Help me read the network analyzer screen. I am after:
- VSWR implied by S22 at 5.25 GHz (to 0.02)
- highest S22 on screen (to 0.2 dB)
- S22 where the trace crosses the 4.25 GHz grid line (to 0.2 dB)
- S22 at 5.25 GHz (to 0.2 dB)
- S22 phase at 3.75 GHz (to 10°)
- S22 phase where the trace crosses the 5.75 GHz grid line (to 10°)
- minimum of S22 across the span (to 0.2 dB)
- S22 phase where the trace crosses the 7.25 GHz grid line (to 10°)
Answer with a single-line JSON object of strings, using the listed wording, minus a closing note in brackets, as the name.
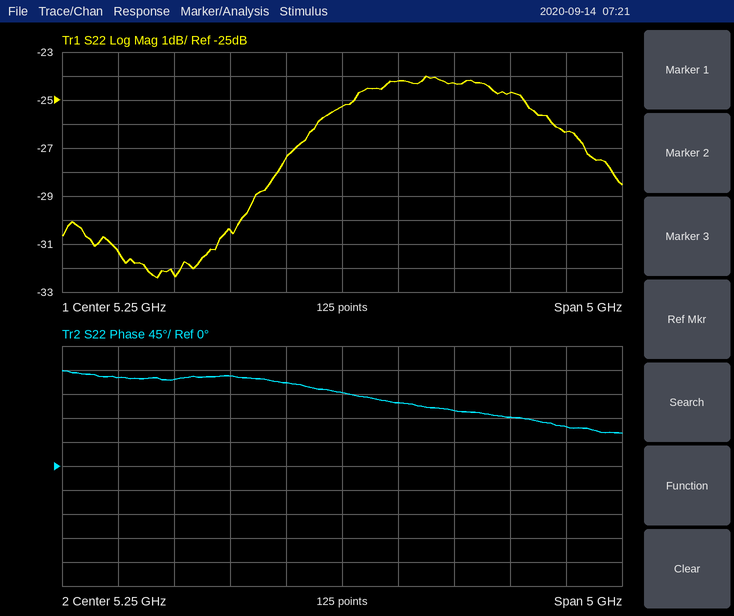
{"VSWR implied by S22 at 5.25 GHz": "1.12", "highest S22 on screen": "-24.0 dB", "S22 where the trace crosses the 4.25 GHz grid line": "-30.4 dB", "S22 at 5.25 GHz": "-25.2 dB", "S22 phase at 3.75 GHz": "160°", "S22 phase where the trace crosses the 5.75 GHz grid line": "120°", "minimum of S22 across the span": "-32.4 dB", "S22 phase where the trace crosses the 7.25 GHz grid line": "70°"}
